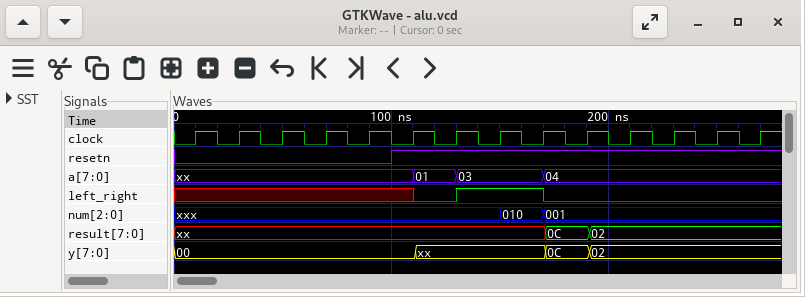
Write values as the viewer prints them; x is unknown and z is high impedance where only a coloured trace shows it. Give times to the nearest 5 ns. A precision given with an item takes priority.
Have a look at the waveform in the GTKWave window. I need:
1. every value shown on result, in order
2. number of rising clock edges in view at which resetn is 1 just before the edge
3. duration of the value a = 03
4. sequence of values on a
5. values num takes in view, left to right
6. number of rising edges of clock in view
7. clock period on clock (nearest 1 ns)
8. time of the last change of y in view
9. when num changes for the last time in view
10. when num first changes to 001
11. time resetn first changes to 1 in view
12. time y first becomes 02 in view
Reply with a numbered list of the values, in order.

1. xx, 0C, 02
2. 9
3. 40 ns
4. xx, 01, 03, 04
5. xxx, 010, 001
6. 14
7. 20 ns
8. 190 ns
9. 170 ns
10. 170 ns
11. 100 ns
12. 190 ns
